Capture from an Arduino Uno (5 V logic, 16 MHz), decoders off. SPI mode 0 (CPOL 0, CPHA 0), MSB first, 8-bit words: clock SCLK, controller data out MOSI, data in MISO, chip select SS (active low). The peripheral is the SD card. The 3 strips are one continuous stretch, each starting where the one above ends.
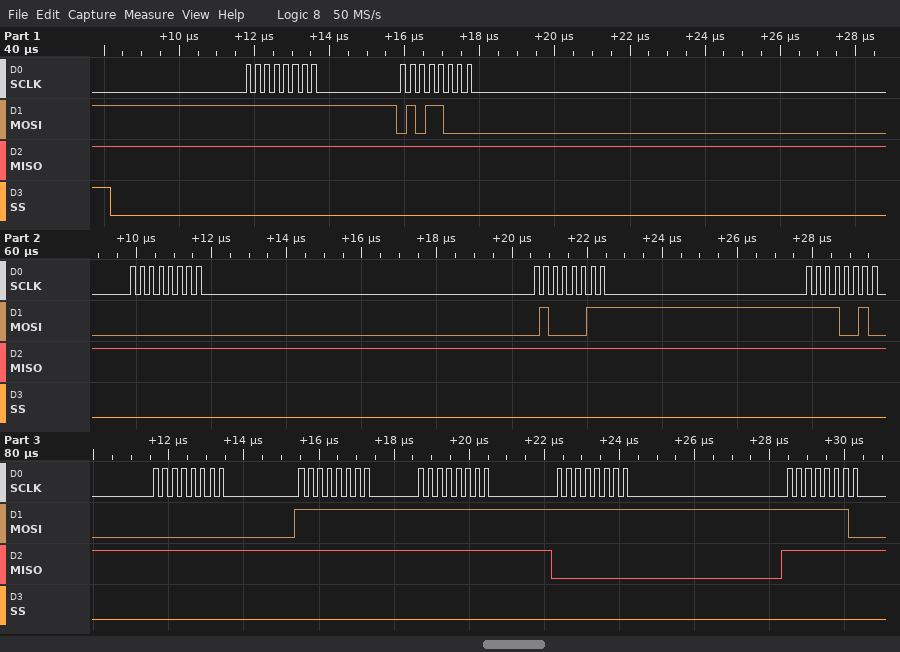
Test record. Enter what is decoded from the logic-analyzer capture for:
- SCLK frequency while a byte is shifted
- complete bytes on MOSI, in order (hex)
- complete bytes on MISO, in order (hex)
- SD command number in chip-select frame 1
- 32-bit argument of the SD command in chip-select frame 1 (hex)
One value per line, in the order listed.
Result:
4 MHz
0xFF 0x58 0x00 0x43 0xF2 0x00 0xFF 0xFF 0xFF 0xFE
0xFF 0xFF 0xFF 0xFF 0xFF 0xFF 0xFF 0xFF 0x00 0xFF
CMD24
0x0043F200
